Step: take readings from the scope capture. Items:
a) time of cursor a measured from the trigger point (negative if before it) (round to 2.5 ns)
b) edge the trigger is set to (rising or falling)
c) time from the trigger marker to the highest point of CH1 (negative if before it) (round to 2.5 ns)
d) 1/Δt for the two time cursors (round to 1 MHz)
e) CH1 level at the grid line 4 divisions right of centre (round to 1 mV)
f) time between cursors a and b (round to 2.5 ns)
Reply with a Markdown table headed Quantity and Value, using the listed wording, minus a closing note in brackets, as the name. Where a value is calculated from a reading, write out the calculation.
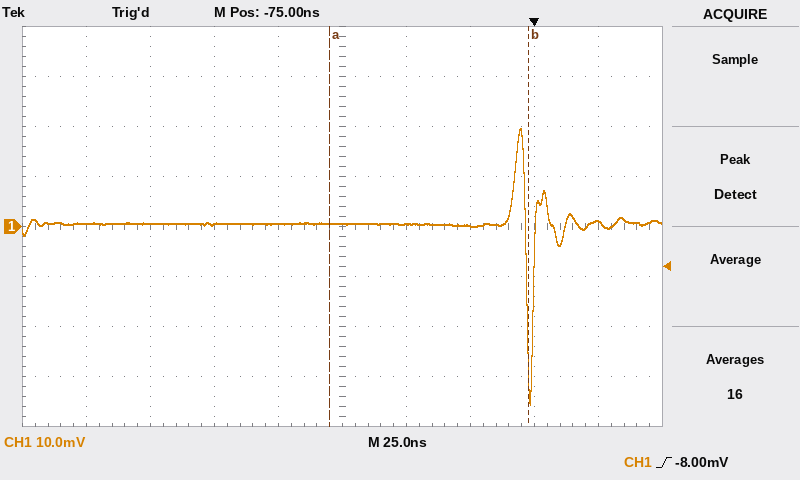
| Quantity | Value |
|---|---|
| time of cursor a measured from the trigger point (negative if before it) | -80.0 ns |
| edge the trigger is set to | rising |
| time from the trigger marker to the highest point of CH1 (negative if before it) | -5.0 ns |
| 1/Δt for the two time cursors | 1 / 77.5 ns ≈ 13 MHz |
| CH1 level at the grid line 4 divisions right of centre | 1 mV |
| time between cursors a and b | 77.5 ns |
